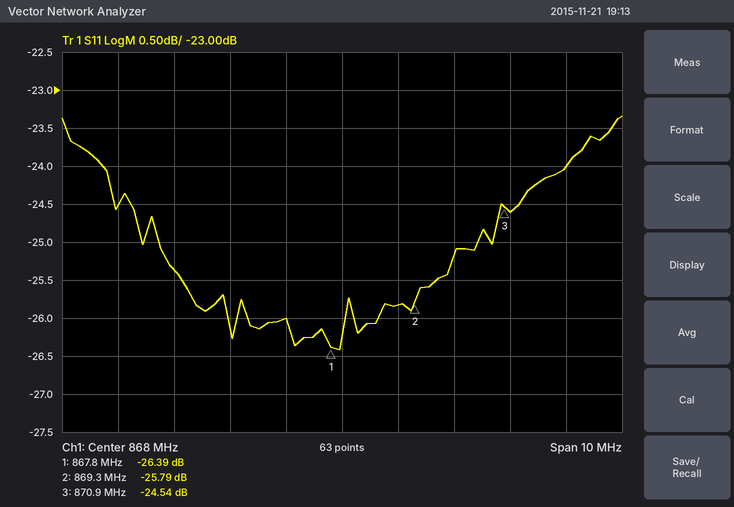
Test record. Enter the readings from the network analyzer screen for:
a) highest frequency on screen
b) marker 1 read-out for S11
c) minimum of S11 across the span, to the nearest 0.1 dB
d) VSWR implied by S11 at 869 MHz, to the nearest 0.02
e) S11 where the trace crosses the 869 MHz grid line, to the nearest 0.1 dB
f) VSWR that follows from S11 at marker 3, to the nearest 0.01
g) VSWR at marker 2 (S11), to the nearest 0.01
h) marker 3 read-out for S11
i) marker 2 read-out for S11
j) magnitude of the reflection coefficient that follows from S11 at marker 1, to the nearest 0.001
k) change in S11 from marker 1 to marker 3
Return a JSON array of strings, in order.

["873 MHz", "-26.39 dB", "-26.4 dB", "1.10", "-25.8 dB", "1.13", "1.11", "-24.54 dB", "-25.79 dB", "0.048", "1.85 dB"]
